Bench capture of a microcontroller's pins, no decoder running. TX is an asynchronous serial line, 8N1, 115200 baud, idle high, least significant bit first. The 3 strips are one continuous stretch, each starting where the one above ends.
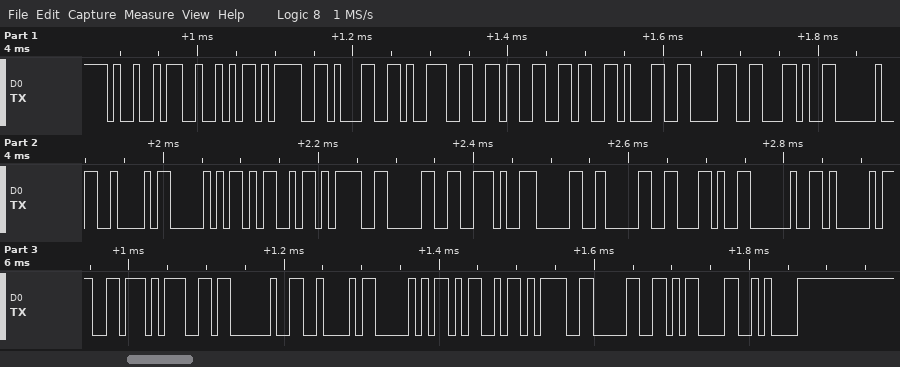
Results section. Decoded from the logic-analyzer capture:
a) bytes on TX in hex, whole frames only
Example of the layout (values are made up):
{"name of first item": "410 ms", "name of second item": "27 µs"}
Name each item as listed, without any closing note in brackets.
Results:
{"bytes on TX in hex, whole frames only": "0x49 0x52 0x3D 0x31 0x39 0x36 0x36 0x31 0x38 0x2C 0x20 0x42 0x50 0x4D 0x3D 0x30 0x2E 0x30 0x30 0x2C 0x20 0x41 0x76 0x67 0x20 0x42 0x50 0x4D 0x3D 0x30 0x0D 0x0A"}
